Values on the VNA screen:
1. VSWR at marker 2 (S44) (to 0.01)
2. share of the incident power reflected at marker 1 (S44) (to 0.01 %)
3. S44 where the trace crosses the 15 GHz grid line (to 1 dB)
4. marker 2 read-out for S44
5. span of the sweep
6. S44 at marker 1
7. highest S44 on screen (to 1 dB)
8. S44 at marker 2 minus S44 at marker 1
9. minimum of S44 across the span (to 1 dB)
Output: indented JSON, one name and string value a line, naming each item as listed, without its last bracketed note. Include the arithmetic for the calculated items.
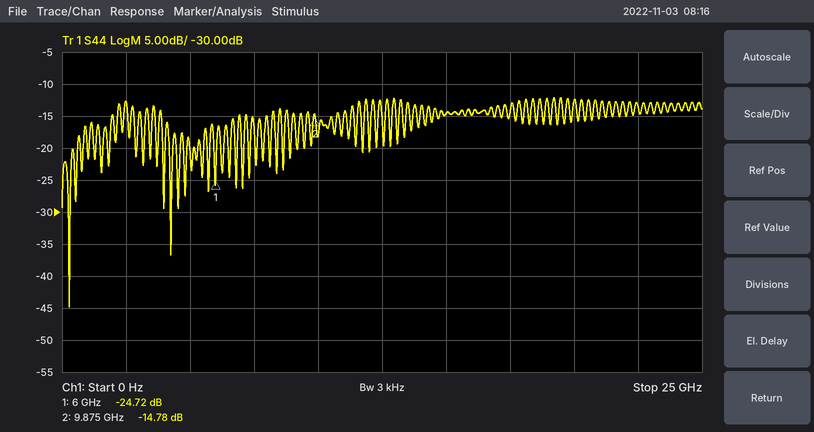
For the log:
{
  "VSWR at marker 2 (S44)": "(1 + 0.1824)/(1 − 0.1824) ≈ 1.45",
  "share of the incident power reflected at marker 1 (S44)": "10^(-24.72/10) ≈ 0.34 %",
  "S44 where the trace crosses the 15 GHz grid line": "-15 dB",
  "marker 2 read-out for S44": "-14.78 dB",
  "span of the sweep": "25 GHz",
  "S44 at marker 1": "-24.72 dB",
  "highest S44 on screen": "-12 dB",
  "S44 at marker 2 minus S44 at marker 1": "-14.78 − (-24.72) = 9.94 dB",
  "minimum of S44 across the span": "-45 dB"
}
